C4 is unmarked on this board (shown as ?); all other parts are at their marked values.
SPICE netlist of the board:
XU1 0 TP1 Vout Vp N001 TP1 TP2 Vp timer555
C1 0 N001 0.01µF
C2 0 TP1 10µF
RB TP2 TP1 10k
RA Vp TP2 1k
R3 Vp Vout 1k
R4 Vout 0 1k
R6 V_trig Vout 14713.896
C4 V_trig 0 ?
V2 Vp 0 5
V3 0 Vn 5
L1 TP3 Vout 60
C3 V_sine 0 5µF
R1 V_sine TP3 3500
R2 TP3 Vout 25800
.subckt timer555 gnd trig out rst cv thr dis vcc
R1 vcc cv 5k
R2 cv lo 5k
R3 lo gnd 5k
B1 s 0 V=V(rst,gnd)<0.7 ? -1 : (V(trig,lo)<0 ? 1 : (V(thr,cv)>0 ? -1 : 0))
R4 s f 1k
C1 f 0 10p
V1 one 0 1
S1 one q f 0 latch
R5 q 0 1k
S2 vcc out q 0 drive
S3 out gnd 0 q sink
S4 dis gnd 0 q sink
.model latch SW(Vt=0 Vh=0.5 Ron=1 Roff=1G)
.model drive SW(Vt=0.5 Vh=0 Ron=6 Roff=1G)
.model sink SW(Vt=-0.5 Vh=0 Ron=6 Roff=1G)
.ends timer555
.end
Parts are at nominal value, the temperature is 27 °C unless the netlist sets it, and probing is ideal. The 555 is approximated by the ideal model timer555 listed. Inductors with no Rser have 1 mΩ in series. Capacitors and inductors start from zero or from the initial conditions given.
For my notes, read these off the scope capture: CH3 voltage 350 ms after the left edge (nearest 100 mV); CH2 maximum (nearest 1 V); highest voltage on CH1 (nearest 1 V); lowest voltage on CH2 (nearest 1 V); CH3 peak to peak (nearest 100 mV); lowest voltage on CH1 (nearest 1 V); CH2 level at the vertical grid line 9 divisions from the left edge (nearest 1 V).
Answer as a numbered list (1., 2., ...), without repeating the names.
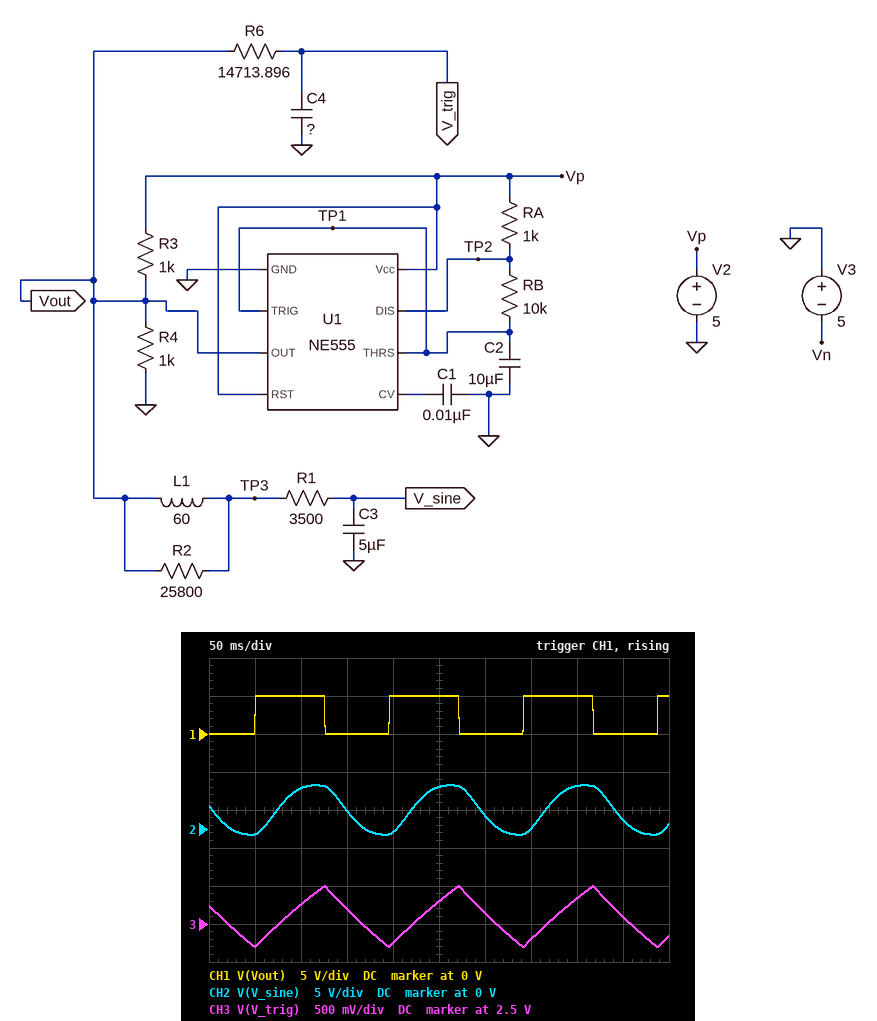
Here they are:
1. 2.3 V
2. 6 V
3. 5 V
4. -1 V
5. 800 mV
6. 0 V
7. 1 V
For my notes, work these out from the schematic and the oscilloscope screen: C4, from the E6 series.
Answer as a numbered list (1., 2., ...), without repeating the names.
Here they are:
1. 15 µF
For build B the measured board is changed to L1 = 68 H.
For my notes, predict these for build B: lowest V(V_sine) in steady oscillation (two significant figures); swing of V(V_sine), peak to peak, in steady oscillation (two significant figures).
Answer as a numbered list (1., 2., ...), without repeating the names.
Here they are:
1. -870 mV
2. 6.7 V
